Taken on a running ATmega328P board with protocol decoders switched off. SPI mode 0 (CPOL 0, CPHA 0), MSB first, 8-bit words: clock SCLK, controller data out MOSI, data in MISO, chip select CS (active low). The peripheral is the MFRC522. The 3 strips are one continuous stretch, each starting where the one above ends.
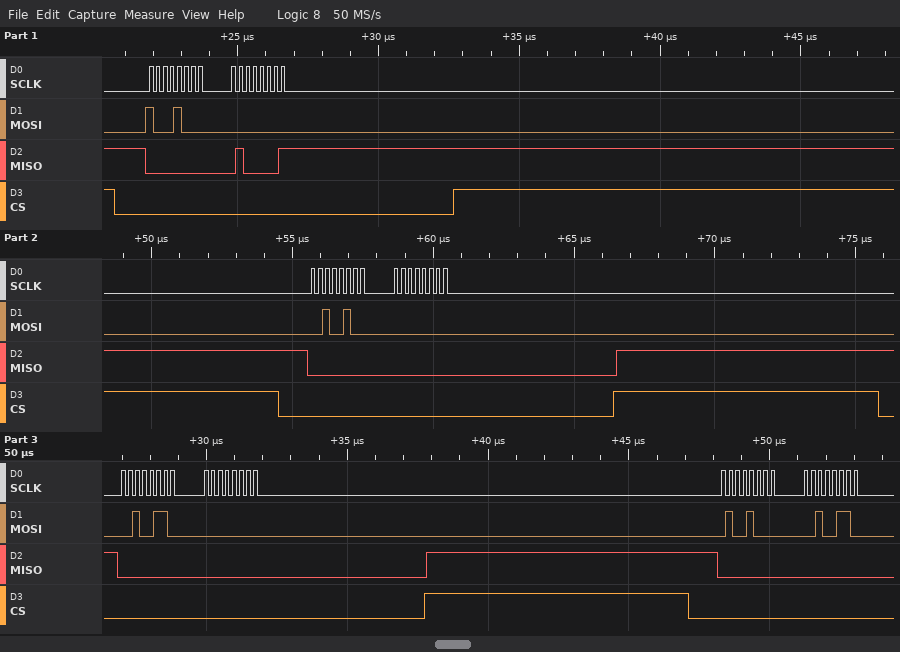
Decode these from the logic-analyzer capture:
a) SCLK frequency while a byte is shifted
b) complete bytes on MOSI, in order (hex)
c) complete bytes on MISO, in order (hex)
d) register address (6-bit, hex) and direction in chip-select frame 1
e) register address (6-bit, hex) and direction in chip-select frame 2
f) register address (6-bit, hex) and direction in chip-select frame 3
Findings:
4 MHz
88 00 24 00 26 00 48 26
00 41 00 00 00 00 00 00
0x04 read
0x12 write
0x13 write
